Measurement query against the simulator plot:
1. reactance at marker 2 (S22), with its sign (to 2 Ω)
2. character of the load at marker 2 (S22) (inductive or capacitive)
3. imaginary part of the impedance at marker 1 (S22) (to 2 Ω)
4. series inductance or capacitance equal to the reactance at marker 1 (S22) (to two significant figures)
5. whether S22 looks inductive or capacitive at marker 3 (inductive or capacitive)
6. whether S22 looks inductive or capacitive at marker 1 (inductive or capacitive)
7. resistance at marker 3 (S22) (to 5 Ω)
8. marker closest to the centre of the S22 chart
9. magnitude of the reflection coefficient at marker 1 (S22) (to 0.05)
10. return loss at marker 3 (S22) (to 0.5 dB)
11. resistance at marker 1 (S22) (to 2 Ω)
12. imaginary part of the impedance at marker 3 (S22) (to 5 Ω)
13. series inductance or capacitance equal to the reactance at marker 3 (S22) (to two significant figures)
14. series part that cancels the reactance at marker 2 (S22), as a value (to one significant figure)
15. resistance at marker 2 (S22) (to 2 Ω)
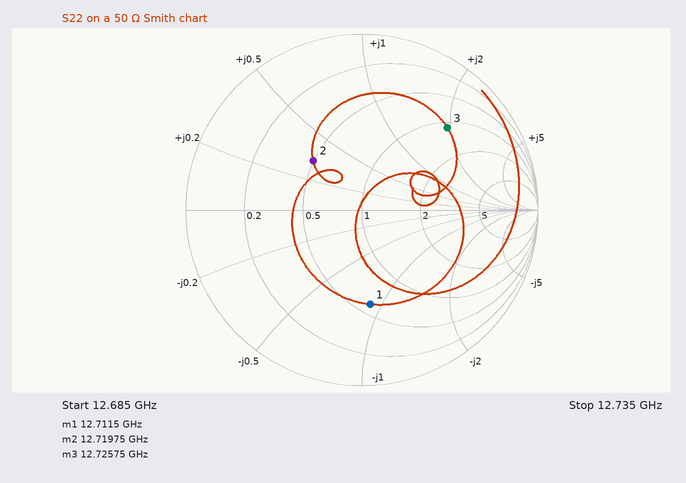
+16 Ω
inductive
-44 Ω
280 fF
inductive
capacitive
55 Ω
marker 2
0.55
3.5 dB
30 Ω
+95 Ω
1.2 nH
800 fF
24 Ω
